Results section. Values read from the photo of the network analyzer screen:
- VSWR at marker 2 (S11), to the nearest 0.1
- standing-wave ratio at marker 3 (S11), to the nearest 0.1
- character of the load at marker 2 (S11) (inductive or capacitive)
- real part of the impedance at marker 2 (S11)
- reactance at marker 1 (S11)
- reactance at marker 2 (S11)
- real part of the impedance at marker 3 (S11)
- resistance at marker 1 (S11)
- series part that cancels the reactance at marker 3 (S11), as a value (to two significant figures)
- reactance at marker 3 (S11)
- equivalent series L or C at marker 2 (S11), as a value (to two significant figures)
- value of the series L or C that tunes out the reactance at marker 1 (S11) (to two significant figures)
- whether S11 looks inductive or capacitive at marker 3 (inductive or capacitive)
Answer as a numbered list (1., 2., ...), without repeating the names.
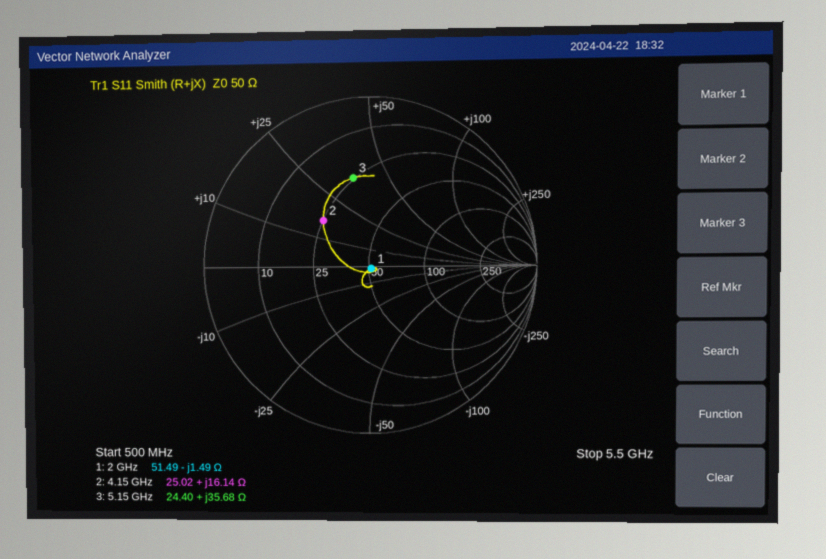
1. 2.3
2. 3.3
3. inductive
4. 25.02 Ω
5. -1.49 Ω
6. +16.14 Ω
7. 24.40 Ω
8. 51.49 Ω
9. 870 fF
10. +35.68 Ω
11. 620 pH
12. 120 pH
13. inductive
